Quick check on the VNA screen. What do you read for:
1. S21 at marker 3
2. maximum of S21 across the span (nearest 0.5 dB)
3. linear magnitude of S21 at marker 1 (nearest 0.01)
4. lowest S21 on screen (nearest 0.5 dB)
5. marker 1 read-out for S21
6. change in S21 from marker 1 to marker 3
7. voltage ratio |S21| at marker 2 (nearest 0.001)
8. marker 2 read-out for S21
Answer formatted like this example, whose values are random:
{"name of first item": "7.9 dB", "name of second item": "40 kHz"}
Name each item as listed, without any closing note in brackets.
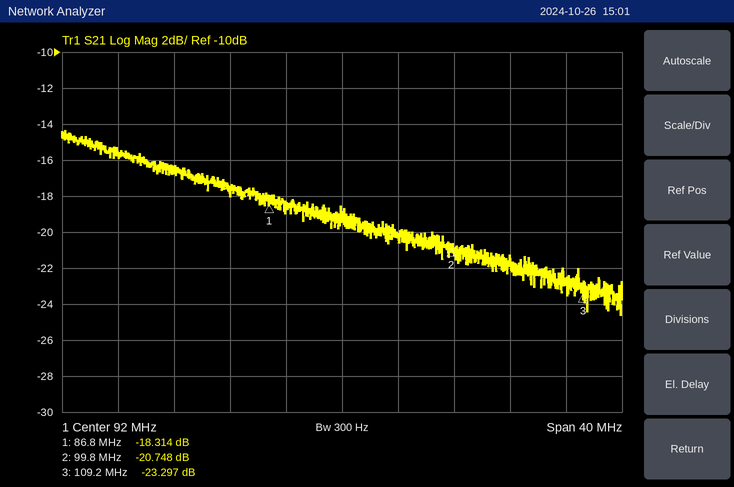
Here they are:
{"S21 at marker 3": "-23.297 dB", "maximum of S21 across the span": "-14.5 dB", "linear magnitude of S21 at marker 1": "0.12", "lowest S21 on screen": "-24.5 dB", "marker 1 read-out for S21": "-18.314 dB", "change in S21 from marker 1 to marker 3": "-4.983 dB", "voltage ratio |S21| at marker 2": "0.092", "marker 2 read-out for S21": "-20.748 dB"}
